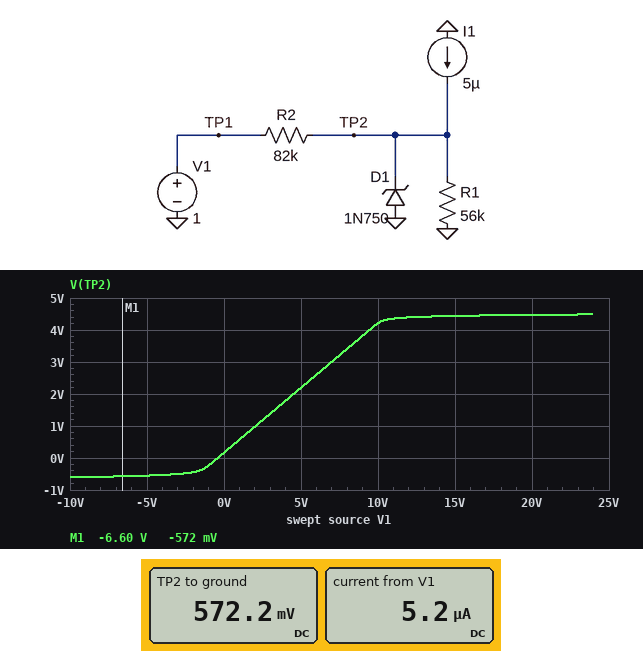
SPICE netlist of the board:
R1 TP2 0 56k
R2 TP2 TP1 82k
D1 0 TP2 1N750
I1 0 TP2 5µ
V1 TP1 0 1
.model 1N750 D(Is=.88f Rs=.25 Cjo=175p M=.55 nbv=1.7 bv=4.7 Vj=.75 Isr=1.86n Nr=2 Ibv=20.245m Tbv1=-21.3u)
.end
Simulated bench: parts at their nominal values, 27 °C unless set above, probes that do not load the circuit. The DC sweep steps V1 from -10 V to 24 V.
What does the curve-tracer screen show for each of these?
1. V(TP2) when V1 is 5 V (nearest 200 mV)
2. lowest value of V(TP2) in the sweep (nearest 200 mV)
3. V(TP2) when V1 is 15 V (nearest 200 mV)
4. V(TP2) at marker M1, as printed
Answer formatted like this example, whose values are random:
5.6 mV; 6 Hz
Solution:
2.2 V; -600 mV; 4.4 V; -572 mV
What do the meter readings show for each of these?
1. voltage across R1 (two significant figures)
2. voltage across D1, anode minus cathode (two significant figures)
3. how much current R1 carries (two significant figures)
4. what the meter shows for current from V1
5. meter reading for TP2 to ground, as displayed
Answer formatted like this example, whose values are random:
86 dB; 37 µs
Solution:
570 mV; -570 mV; 10 µA; 5.2 µA; 572.2 mV
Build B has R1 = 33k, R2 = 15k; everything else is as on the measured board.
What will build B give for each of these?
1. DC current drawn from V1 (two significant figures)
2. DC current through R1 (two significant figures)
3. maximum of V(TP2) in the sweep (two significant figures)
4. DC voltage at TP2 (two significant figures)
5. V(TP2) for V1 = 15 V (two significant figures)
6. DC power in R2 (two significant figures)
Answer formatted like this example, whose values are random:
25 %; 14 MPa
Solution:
17 µA; 22 µA; 4.6 V; 740 mV; 4.5 V; 4.5 µW
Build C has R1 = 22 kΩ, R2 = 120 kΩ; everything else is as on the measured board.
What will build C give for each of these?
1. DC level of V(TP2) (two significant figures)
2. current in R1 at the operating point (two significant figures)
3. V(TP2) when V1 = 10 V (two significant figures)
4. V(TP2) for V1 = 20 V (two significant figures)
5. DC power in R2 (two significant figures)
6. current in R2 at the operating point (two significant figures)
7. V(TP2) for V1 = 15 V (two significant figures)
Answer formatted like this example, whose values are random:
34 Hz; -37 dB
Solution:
250 mV; 11 µA; 1.6 V; 3.2 V; 4.7 µW; 6.3 µA; 2.4 V
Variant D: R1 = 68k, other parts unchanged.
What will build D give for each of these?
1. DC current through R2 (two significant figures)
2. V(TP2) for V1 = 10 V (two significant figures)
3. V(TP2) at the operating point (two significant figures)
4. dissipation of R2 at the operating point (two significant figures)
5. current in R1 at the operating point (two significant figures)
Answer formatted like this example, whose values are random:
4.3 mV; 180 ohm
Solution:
4.4 µA; 4.4 V; 640 mV; 1.6 µW; 9.4 µA
